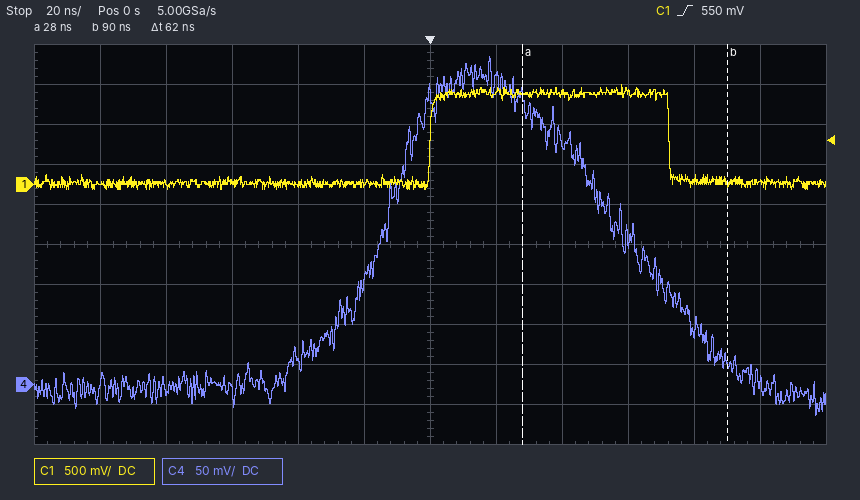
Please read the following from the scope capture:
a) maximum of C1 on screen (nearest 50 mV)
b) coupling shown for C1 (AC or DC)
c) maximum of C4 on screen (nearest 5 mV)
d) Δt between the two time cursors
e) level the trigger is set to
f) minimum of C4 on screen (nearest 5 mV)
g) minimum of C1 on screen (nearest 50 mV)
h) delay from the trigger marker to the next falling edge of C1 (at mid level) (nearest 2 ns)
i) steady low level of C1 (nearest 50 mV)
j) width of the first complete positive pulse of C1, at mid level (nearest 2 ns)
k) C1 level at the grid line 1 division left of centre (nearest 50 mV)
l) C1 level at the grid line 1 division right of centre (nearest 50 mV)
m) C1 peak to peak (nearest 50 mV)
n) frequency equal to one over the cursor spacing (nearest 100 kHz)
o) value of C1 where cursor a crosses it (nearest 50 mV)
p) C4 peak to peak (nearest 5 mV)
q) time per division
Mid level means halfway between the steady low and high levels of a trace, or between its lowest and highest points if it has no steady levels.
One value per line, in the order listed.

1.25 V
DC
410 mV
62 ns
550 mV
-40 mV
-50 mV
72 ns
0 mV
72 ns
0 mV
1.15 V
1.30 V
16.1 MHz
1.15 V
450 mV
20 ns
